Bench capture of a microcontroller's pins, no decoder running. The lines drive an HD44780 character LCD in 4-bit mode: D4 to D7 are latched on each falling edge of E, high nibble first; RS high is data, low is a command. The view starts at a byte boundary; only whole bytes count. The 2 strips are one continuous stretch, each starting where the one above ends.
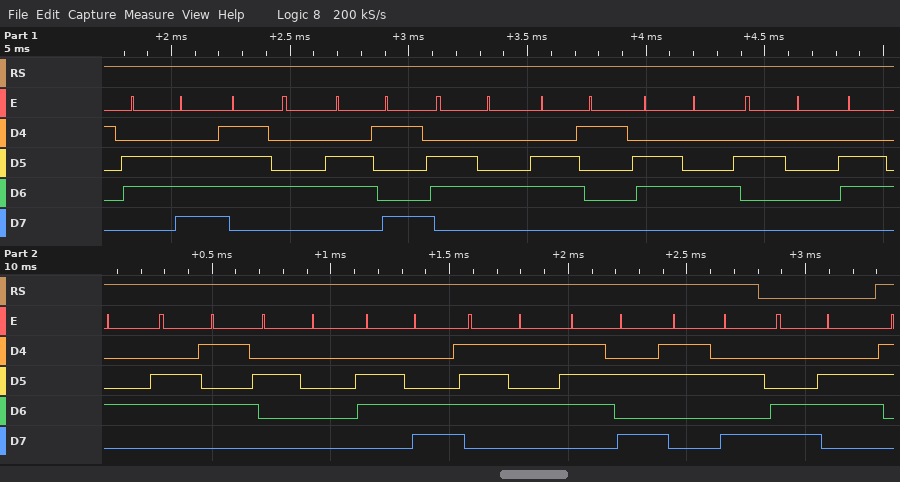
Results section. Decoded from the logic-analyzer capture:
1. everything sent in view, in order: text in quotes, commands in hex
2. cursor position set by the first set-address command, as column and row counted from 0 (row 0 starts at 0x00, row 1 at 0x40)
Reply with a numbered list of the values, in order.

1. "ntidad de luz:" 0xC6
2. column 6, row 1
